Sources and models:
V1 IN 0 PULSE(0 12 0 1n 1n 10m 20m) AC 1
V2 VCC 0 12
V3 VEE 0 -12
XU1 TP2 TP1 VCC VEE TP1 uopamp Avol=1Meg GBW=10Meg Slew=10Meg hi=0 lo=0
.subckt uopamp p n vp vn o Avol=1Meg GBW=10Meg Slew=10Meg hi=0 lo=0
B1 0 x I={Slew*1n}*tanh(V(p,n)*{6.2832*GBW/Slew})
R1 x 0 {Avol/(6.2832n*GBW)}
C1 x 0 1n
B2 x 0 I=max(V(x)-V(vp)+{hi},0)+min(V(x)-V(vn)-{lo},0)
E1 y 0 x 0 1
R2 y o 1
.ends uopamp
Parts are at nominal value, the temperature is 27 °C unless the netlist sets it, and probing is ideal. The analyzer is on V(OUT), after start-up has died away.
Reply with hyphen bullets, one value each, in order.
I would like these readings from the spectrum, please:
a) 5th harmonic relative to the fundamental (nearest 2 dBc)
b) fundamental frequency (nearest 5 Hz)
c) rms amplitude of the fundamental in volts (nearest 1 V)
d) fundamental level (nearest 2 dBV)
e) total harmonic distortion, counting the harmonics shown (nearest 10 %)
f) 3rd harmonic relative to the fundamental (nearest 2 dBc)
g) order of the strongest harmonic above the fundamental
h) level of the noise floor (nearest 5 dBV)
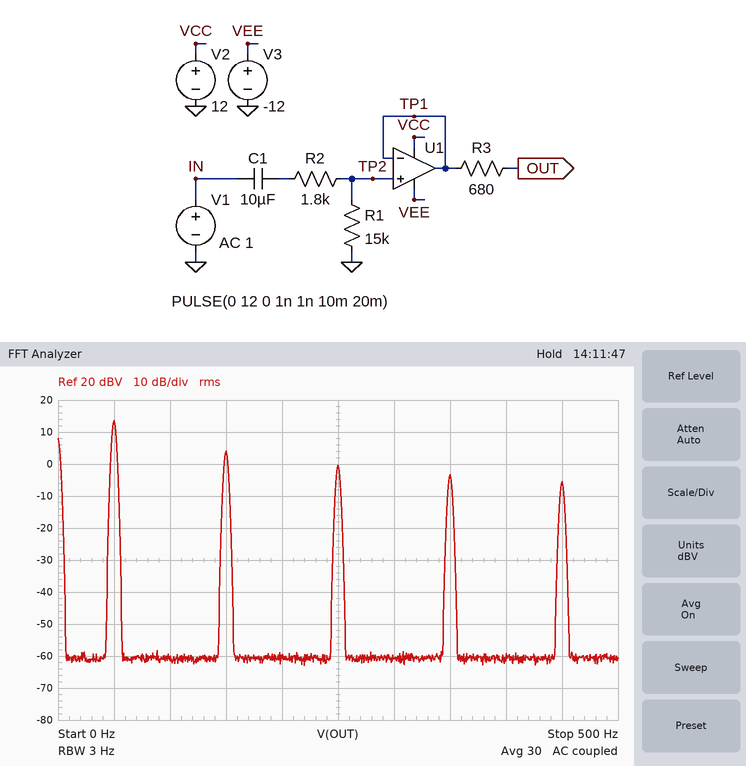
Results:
- -14 dBc
- 50 Hz
- 5 V
- 14 dBV
- 40 %
- -10 dBc
- 3
- -60 dBV
